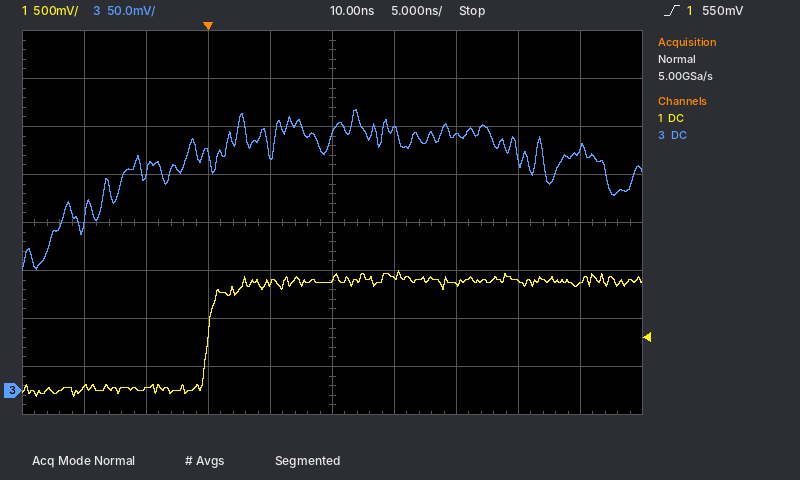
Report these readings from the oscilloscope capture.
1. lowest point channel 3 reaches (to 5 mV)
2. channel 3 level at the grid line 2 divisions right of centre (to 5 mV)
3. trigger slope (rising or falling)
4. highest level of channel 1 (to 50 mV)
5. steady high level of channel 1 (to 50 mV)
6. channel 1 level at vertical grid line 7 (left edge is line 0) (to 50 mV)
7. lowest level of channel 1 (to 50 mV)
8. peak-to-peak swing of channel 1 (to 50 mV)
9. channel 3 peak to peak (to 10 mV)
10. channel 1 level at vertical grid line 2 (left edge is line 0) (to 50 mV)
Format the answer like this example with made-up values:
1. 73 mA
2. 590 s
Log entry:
1. 125 mV
2. 265 mV
3. rising
4. 1.25 V
5. 1.15 V
6. 1.10 V
7. -50 mV
8. 1.30 V
9. 170 mV
10. 0 mV
